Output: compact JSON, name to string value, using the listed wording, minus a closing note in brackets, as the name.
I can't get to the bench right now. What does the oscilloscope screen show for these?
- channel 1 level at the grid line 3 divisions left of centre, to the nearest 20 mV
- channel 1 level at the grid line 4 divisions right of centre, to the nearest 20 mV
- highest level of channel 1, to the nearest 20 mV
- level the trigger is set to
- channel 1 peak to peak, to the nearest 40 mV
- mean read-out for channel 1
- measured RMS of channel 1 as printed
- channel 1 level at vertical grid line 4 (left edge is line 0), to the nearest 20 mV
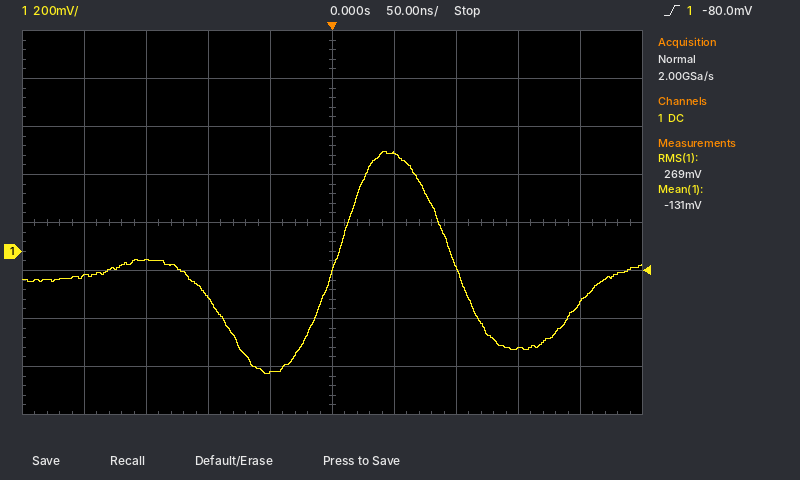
{"channel 1 level at the grid line 3 divisions left of centre, to the nearest 20 mV": "-40 mV", "channel 1 level at the grid line 4 divisions right of centre, to the nearest 20 mV": "-220 mV", "highest level of channel 1, to the nearest 20 mV": "420 mV", "level the trigger is set to": "-80.0 mV", "channel 1 peak to peak, to the nearest 40 mV": "920 mV", "mean read-out for channel 1": "-131 mV", "measured RMS of channel 1 as printed": "269 mV", "channel 1 level at vertical grid line 4 (left edge is line 0), to the nearest 20 mV": "-500 mV"}
